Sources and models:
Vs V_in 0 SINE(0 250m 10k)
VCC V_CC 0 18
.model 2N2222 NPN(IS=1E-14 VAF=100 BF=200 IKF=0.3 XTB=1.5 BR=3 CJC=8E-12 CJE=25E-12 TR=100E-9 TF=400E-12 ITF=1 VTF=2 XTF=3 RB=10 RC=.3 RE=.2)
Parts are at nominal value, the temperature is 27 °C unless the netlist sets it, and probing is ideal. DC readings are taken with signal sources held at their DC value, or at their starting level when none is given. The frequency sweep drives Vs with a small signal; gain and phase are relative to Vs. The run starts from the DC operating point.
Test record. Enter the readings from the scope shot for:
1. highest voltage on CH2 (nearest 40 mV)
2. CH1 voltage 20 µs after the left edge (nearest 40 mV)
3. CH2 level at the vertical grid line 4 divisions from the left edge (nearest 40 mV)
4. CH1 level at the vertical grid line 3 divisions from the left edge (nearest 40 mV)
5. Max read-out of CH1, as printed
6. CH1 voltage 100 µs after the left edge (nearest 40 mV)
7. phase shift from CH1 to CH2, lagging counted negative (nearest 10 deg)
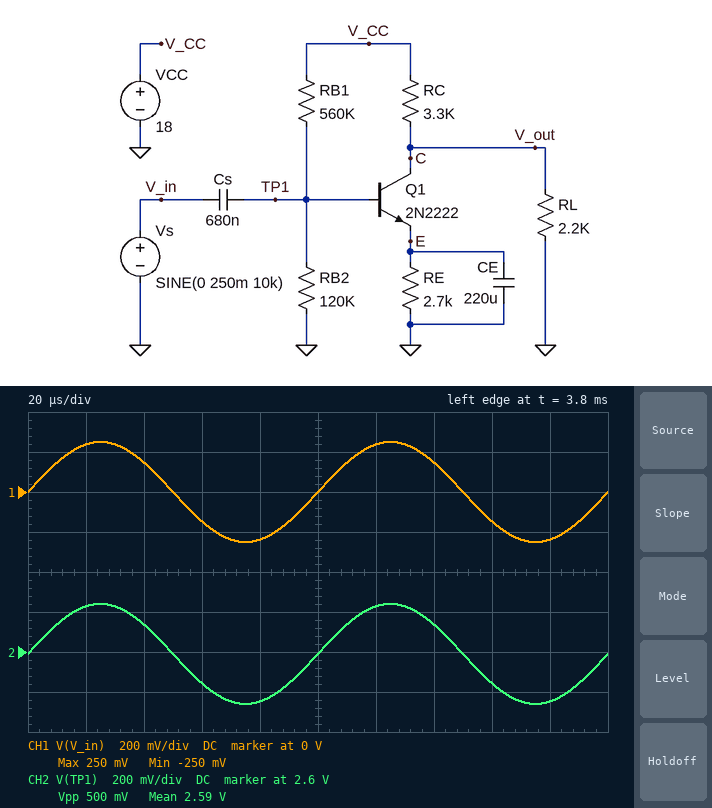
2.84 V
240 mV
2.36 V
-160 mV
250 mV
0 V
0 deg
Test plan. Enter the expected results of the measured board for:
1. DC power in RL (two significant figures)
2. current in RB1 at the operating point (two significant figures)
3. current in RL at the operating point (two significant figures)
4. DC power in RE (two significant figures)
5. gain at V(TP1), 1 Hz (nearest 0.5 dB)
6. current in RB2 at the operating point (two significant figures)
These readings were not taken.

17 mW
27 µA
2.8 mA
1.7 mW
-11.5 dB
23 µA
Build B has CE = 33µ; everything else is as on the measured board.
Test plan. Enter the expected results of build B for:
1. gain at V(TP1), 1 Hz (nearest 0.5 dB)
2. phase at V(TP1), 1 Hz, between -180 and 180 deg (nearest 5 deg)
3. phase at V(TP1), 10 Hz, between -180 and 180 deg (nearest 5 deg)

-9.5 dB
65 deg
15 deg
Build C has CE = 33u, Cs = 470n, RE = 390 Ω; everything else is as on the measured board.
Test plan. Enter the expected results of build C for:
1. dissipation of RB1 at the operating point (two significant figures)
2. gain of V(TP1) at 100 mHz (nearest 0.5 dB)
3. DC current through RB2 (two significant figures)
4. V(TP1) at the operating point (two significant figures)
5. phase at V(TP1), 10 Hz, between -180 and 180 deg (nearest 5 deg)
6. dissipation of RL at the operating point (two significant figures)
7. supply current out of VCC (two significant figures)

470 µW
-38.0 dB
15 µA
1.8 V
30 deg
5.5 mW
4.4 mA
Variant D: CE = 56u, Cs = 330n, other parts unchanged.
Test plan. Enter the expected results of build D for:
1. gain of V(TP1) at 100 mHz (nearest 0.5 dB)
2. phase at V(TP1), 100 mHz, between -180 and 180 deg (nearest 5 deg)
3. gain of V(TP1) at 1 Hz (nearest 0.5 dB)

-35.0 dB
90 deg
-15.5 dB
